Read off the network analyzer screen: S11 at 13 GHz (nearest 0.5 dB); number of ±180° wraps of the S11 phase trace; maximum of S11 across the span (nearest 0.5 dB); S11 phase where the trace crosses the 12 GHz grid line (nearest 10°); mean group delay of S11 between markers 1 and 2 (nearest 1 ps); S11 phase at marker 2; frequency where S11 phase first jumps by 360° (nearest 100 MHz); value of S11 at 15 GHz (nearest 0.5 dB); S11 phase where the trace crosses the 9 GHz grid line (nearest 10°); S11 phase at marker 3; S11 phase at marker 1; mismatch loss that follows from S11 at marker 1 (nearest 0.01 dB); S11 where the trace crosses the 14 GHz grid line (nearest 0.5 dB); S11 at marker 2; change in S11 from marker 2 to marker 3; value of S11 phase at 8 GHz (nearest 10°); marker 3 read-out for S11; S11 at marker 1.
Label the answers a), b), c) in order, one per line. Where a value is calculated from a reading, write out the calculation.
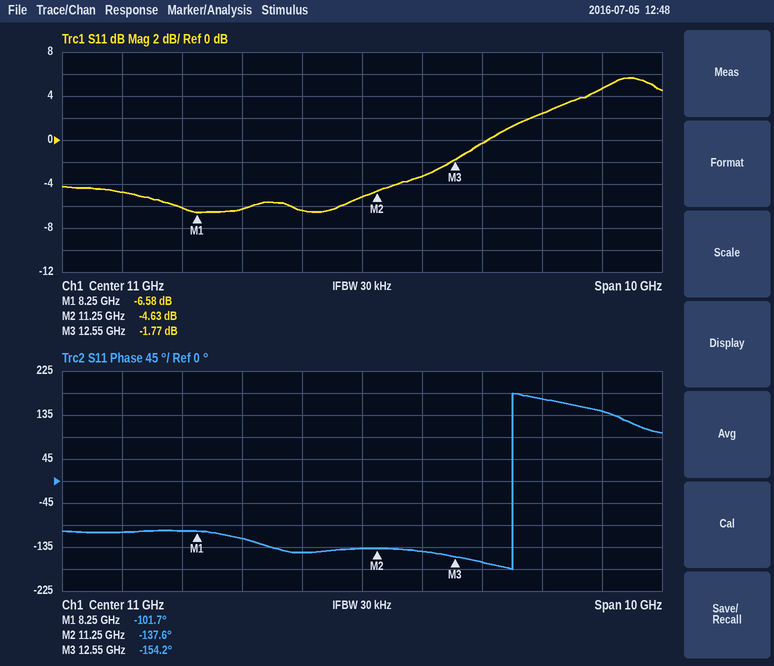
a) -0.5 dB
b) 1
c) 5.5 dB
d) -140°
e) −(-137.6° − (-101.7°))/(360° × 3 GHz) ≈ 33 ps
f) -137.6°
g) 13.5 GHz
h) 4.5 dB
i) -120°
j) -154.2°
k) -101.7°
l) −10 log10(1 − 10^(-6.58/10)) ≈ 1.08 dB
m) 2.5 dB
n) -4.63 dB
o) -1.77 − (-4.63) = 2.86 dB
p) -100°
q) -1.77 dB
r) -6.58 dB
